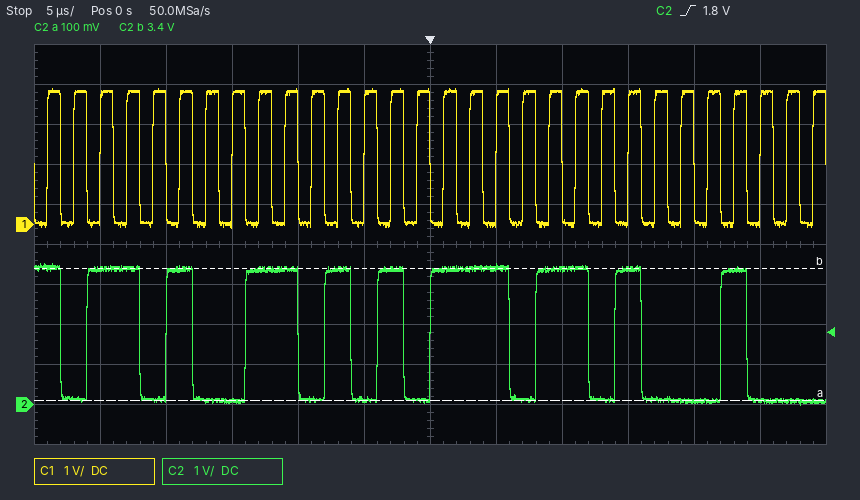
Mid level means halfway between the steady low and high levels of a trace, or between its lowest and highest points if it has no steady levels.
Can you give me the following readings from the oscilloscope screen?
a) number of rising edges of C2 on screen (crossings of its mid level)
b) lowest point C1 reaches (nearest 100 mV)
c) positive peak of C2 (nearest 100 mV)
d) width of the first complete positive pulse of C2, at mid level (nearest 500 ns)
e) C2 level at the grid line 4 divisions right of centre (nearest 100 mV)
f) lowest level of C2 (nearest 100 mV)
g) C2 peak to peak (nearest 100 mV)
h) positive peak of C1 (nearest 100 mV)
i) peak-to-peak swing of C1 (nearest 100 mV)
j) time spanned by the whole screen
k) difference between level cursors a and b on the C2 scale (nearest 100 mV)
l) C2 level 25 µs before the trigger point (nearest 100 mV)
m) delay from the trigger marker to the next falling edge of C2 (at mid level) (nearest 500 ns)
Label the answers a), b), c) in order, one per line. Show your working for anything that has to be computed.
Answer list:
a) 9
b) -100 mV
c) 3.5 V
d) 4.0 µs
e) 100 mV
f) 0.0 V
g) 3.5 V − (0.0 V) = 3.5 V
h) 3.4 V
i) 3.4 V − (-100 mV) = 3.5 V
j) 60 µs
k) 3.3 V
l) 3.4 V
m) 6.0 µs
